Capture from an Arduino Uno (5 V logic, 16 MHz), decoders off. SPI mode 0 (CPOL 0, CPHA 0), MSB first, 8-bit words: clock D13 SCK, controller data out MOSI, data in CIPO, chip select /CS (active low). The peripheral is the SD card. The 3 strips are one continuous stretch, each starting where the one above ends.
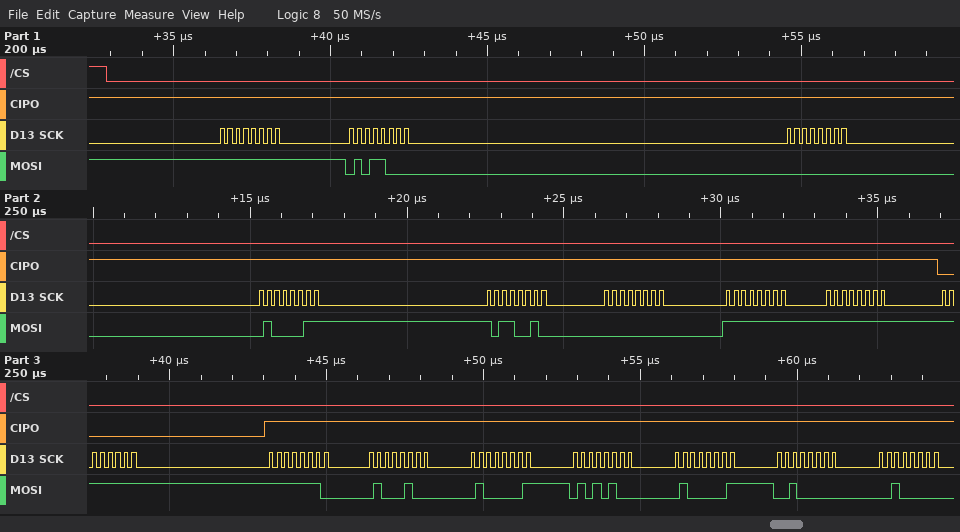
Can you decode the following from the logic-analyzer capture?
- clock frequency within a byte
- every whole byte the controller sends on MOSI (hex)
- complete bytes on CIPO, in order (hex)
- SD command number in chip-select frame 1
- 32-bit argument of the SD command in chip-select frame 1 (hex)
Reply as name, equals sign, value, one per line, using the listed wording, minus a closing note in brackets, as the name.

clock frequency within a byte = 4 MHz
every whole byte the controller sends on MOSI = FF 58 00 43 B2 00 FF FF FF FE 44 41 54 41 20 20
complete bytes on CIPO, in order = FF FF FF FF FF FF FF FF 00 FF FF FF FF FF FF FF
SD command number in chip-select frame 1 = CMD24
32-bit argument of the SD command in chip-select frame 1 = 0x0043B200
